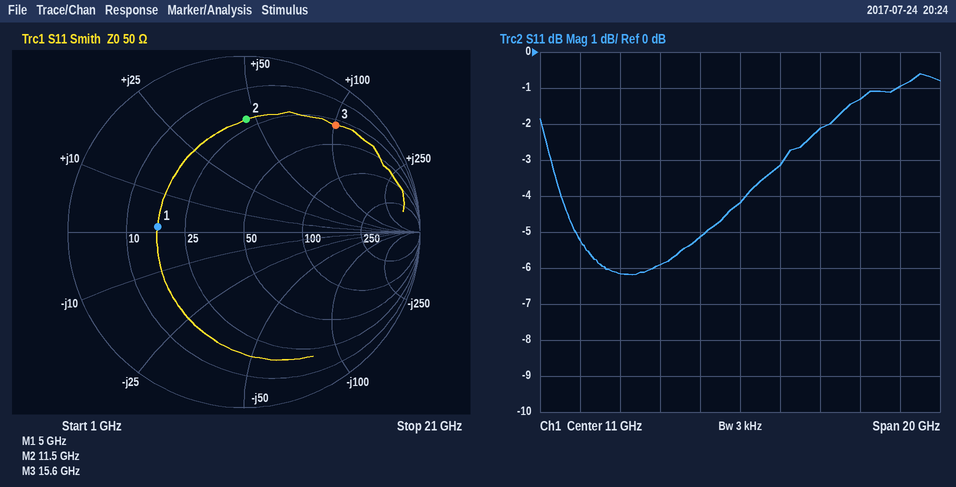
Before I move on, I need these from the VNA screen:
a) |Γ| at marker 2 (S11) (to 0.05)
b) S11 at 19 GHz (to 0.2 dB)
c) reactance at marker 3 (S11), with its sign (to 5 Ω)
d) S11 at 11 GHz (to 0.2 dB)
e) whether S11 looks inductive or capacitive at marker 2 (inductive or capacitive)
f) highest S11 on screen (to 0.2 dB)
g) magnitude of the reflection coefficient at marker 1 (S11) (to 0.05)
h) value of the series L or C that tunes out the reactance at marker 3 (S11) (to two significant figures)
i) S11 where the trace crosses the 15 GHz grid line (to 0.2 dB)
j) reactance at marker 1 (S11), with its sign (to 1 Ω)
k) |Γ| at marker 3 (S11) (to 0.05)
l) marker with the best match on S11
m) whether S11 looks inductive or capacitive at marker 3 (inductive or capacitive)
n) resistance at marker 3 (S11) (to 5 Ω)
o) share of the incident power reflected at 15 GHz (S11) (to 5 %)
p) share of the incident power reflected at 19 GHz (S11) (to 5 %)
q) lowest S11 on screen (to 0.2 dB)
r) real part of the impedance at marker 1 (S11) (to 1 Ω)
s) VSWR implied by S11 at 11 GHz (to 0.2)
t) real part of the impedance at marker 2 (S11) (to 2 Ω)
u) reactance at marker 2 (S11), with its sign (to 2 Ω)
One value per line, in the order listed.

0.65
-1.0 dB
+100 Ω
-4.2 dB
inductive
-0.6 dB
0.50
100 fF
-2.2 dB
+1 Ω
0.80
marker 1
inductive
30 Ω
60 %
80 %
-6.2 dB
17 Ω
4.2
22 Ω
+46 Ω
